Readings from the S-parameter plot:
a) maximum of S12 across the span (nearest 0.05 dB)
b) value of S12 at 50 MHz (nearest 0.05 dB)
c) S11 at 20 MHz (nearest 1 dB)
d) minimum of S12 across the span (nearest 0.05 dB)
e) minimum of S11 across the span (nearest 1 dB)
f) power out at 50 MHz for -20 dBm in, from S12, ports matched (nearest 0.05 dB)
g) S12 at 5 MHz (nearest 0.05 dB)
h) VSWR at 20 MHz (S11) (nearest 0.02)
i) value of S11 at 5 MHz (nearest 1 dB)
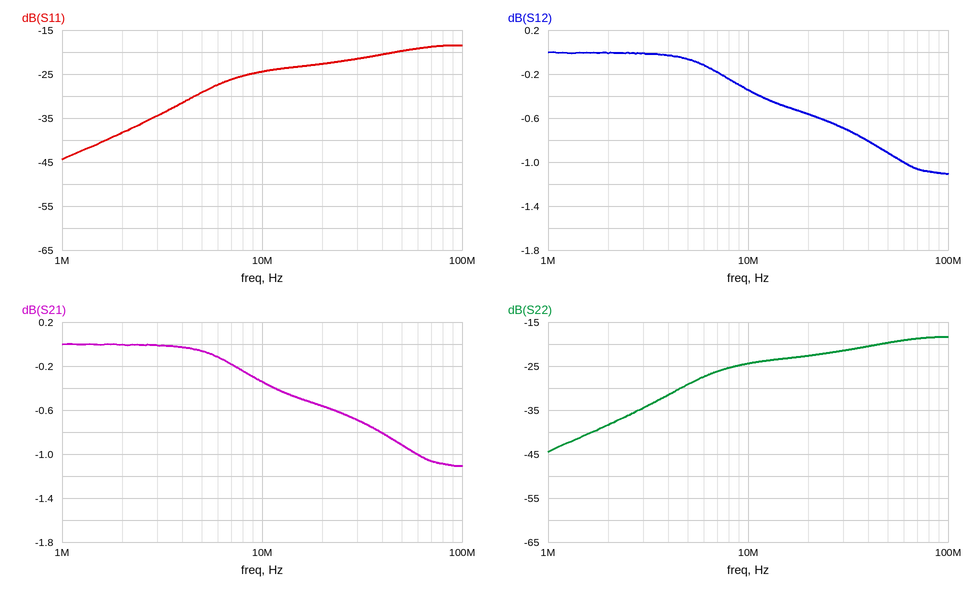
0.00 dB
-0.90 dB
-23 dB
-1.10 dB
-44 dB
-20.90 dBm
-0.05 dB
1.16
-29 dB
